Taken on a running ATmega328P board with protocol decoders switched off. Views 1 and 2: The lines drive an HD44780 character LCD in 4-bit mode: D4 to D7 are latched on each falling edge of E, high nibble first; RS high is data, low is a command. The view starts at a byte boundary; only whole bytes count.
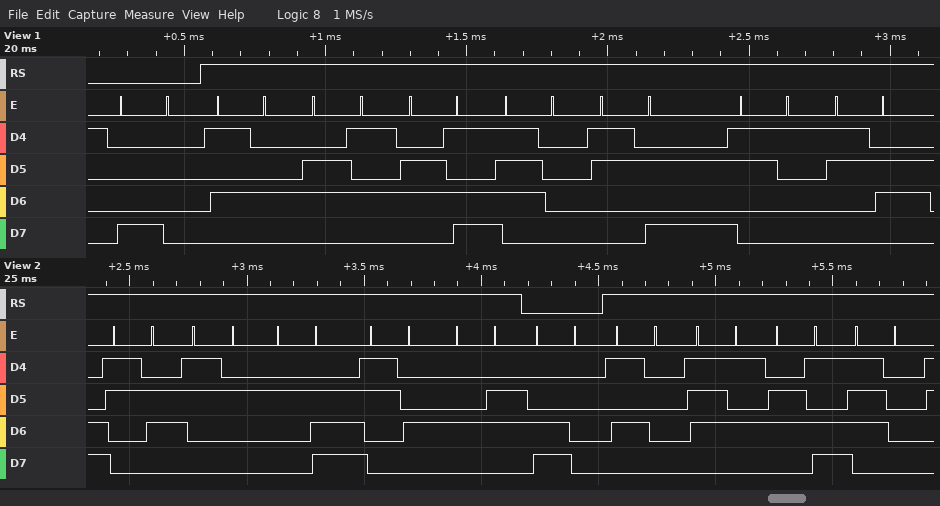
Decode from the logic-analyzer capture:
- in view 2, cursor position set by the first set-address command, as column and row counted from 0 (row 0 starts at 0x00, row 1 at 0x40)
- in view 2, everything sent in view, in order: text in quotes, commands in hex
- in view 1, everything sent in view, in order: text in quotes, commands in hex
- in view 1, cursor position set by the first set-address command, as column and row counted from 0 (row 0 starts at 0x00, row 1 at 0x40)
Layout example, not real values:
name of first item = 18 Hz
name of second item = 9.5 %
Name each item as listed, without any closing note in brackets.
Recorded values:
in view 2, cursor position set by the first set-address command, as column and row counted from 0 = column 0, row 1
in view 2, everything sent in view, in order: text in quotes, commands in hex = "62.4F" 0xC0 "Pump"
in view 1, everything sent in view, in order: text in quotes, commands in hex = 0x80 "Temp:16"
in view 1, cursor position set by the first set-address command, as column and row counted from 0 = column 0, row 0
